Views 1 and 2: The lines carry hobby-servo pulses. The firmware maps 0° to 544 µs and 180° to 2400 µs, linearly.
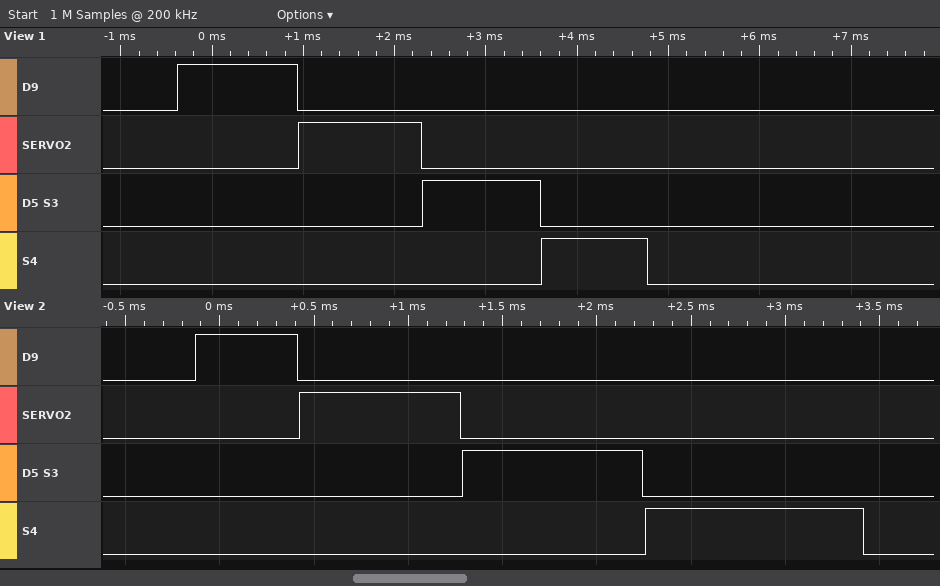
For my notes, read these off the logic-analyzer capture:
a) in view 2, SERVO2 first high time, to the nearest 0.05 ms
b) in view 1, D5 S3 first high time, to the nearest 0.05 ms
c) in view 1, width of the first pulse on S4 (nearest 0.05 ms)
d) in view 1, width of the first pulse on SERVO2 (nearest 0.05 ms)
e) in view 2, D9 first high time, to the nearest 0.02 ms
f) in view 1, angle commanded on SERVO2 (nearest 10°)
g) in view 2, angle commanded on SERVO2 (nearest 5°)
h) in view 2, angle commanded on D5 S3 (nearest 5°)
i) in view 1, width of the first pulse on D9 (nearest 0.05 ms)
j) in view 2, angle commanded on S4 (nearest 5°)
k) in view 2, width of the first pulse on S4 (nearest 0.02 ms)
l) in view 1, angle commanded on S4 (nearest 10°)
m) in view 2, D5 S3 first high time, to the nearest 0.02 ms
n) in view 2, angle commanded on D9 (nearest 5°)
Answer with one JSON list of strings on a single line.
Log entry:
["0.85 ms", "1.30 ms", "1.15 ms", "1.35 ms", "0.54 ms", "80°", "30°", "40°", "1.30 ms", "60°", "1.16 ms", "60°", "0.96 ms", "0°"]
